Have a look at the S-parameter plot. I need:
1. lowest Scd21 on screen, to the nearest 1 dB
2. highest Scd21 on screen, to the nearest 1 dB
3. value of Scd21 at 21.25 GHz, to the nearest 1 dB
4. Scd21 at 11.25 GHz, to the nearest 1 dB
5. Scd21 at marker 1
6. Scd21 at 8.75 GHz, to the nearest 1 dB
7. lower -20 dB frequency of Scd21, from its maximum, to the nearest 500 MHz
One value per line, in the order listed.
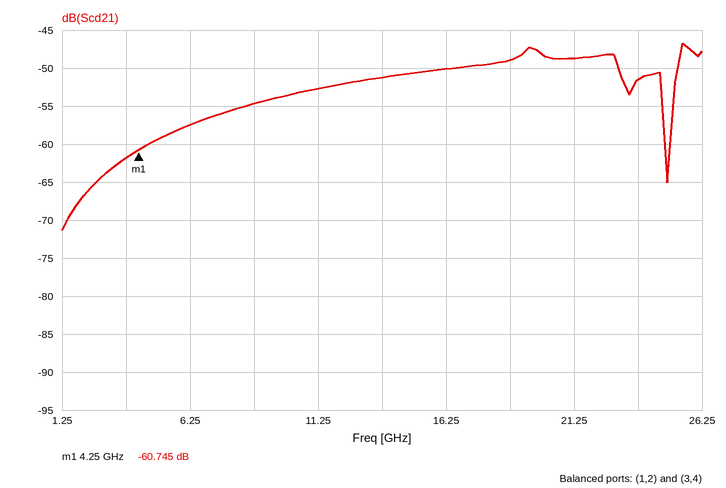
-71 dB
-47 dB
-49 dB
-53 dB
-60.745 dB
-55 dB
2.0 GHz
